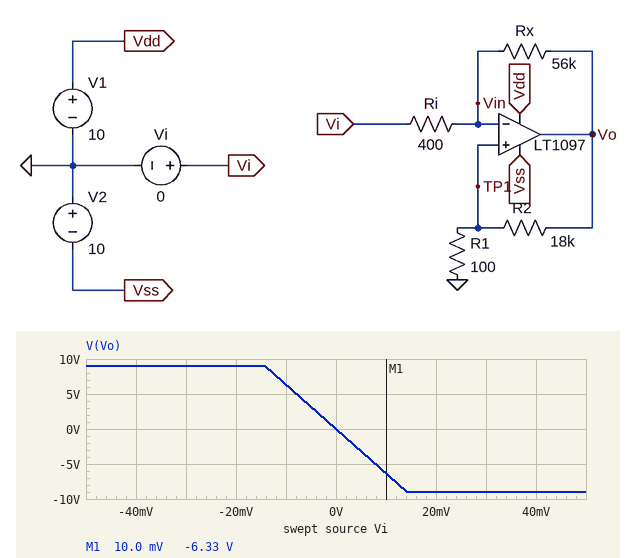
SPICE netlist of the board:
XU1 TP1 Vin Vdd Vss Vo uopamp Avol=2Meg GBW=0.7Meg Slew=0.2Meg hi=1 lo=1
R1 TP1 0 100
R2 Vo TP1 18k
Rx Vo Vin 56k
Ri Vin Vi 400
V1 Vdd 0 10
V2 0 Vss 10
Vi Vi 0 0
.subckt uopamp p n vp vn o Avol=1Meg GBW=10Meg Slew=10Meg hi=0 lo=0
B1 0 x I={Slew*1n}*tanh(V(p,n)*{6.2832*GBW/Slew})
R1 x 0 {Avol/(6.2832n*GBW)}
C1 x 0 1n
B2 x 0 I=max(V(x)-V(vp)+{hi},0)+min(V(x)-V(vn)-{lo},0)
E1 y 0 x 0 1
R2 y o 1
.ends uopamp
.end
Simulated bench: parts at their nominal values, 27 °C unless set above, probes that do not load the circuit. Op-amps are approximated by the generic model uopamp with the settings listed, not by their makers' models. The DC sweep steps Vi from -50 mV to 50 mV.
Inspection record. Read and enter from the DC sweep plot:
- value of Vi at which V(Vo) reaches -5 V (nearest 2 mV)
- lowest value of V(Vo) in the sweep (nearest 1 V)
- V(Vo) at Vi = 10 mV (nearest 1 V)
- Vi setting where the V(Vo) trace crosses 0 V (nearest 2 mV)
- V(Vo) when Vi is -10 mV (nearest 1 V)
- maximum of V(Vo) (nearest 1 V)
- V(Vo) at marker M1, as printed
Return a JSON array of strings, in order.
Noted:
["8 mV", "-9 V", "-6 V", "0 V", "6 V", "9 V", "-6.33 V"]
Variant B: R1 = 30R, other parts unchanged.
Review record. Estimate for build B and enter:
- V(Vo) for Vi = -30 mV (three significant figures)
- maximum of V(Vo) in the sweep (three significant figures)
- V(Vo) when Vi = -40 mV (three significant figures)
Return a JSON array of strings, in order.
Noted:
["5.49 V", "9.00 V", "7.32 V"]
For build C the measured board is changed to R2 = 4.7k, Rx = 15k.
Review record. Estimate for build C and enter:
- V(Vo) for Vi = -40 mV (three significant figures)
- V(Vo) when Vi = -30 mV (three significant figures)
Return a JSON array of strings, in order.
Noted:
["7.58 V", "5.68 V"]
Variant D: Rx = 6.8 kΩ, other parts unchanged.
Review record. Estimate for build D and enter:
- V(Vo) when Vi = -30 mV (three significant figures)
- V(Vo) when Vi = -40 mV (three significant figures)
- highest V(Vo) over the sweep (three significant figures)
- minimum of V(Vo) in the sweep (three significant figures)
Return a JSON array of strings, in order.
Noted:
["566 mV", "755 mV", "944 mV", "-944 mV"]
